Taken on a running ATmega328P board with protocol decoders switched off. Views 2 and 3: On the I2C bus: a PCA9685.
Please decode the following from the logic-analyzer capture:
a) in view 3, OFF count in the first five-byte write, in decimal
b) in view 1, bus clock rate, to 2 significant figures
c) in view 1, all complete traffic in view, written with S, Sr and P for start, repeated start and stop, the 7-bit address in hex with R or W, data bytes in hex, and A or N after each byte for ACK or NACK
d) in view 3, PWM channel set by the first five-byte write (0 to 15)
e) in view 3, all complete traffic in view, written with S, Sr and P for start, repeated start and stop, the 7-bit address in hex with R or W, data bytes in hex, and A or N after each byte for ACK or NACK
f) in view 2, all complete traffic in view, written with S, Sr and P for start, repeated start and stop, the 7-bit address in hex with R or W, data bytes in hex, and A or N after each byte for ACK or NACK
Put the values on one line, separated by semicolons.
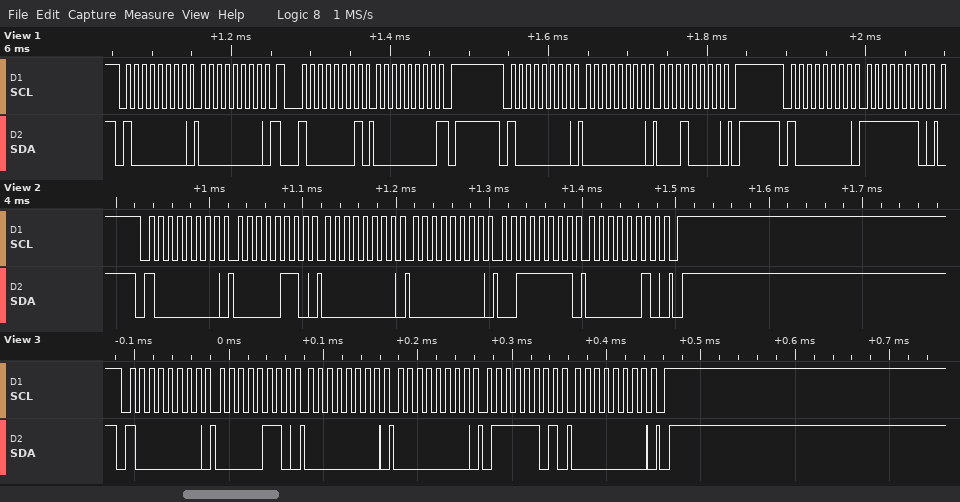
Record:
125; 100 kHz; S 40W A 00 A Sr 40R A 00 N P S 40W A 00 A 10 A P S 40W A FE A; 0; S 40W A 06 A 00 A 00 A 7D A 00 A P; S 40W A 06 A 00 A 00 A 3F A 02 A P
